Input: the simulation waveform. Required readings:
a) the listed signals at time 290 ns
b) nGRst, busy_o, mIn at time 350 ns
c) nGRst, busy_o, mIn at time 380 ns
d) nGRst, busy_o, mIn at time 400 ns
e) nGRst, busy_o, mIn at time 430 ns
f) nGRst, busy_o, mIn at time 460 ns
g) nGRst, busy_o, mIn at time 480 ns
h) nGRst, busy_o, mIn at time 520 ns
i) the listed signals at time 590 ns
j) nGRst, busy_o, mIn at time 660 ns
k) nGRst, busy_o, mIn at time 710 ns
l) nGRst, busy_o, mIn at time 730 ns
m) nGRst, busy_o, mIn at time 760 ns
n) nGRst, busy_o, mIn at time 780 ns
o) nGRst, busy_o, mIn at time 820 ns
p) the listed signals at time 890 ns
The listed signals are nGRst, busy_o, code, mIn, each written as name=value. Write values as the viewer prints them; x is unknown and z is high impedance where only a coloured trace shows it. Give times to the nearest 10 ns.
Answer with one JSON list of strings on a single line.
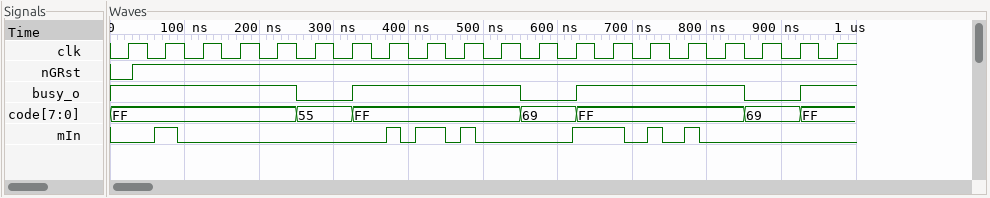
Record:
["nGRst=1, busy_o=0, code=55, mIn=0", "nGRst=1, busy_o=1, mIn=0", "nGRst=1, busy_o=1, mIn=1", "nGRst=1, busy_o=1, mIn=0", "nGRst=1, busy_o=1, mIn=1", "nGRst=1, busy_o=1, mIn=0", "nGRst=1, busy_o=1, mIn=1", "nGRst=1, busy_o=1, mIn=0", "nGRst=1, busy_o=0, code=69, mIn=0", "nGRst=1, busy_o=1, mIn=1", "nGRst=1, busy_o=1, mIn=0", "nGRst=1, busy_o=1, mIn=1", "nGRst=1, busy_o=1, mIn=0", "nGRst=1, busy_o=1, mIn=1", "nGRst=1, busy_o=1, mIn=0", "nGRst=1, busy_o=0, code=69, mIn=0"]
